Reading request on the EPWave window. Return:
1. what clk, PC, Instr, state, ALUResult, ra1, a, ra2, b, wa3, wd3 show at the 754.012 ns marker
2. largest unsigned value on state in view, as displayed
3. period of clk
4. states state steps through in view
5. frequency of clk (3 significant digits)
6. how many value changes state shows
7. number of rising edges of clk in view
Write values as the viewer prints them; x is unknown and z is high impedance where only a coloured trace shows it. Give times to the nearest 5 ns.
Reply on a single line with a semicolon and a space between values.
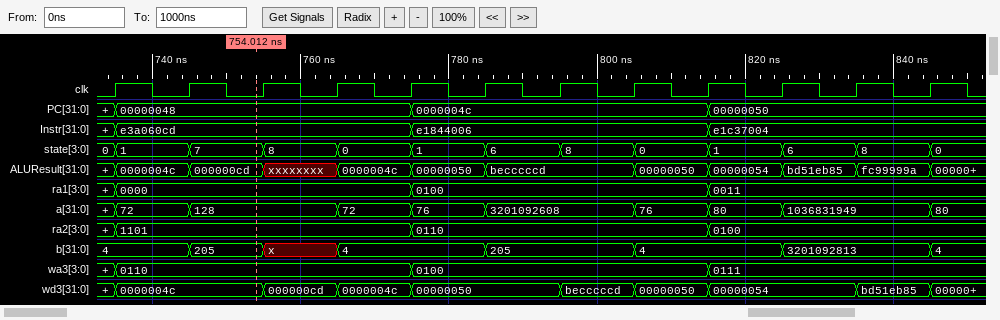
clk=0, PC=00000048, Instr=e3a060cd, state=7, ALUResult=000000cd, ra1=0000, a=128, ra2=1101, b=205, wa3=0110, wd3=0000004c; 8; 10 ns; 0, 1, 7, 8, 0, 1, 6, 8, 0, 1, 6, 8, 0; 100 MHz; 12; 12
